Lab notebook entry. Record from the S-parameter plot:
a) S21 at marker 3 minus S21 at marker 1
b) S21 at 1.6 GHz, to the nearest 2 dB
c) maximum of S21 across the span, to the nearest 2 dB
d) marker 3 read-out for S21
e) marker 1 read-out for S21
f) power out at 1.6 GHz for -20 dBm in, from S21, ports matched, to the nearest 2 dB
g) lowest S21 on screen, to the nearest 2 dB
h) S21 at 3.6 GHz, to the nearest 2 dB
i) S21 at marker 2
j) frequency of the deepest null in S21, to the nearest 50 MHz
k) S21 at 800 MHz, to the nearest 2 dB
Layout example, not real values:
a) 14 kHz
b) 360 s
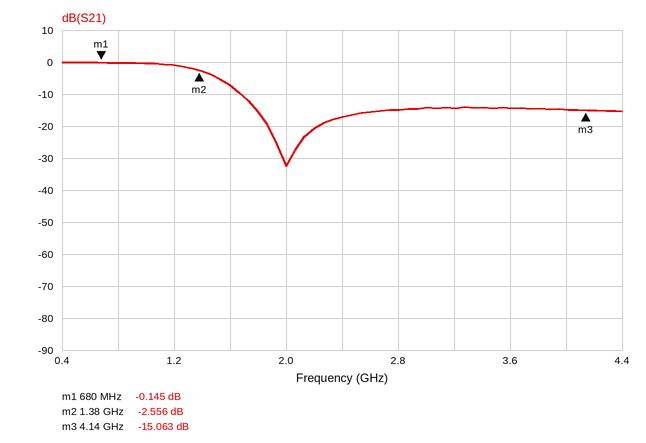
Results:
a) -14.918 dB
b) -8 dB
c) 0 dB
d) -15.063 dB
e) -0.145 dB
f) -28 dBm
g) -32 dB
h) -14 dB
i) -2.556 dB
j) 2.00 GHz
k) 0 dB
